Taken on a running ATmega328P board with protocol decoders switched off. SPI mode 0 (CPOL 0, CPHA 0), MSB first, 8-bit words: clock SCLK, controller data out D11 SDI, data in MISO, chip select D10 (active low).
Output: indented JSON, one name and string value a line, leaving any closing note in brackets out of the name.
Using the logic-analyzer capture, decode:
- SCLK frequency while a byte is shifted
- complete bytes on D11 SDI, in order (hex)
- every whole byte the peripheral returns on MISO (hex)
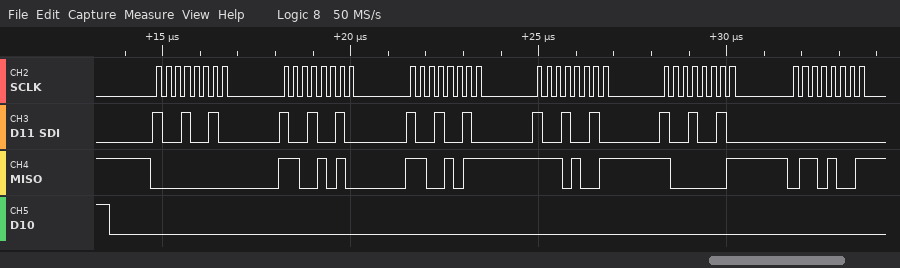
{
  "SCLK frequency while a byte is shifted": "4 MHz",
  "complete bytes on D11 SDI, in order": "92 92 92 92 92 00",
  "every whole byte the peripheral returns on MISO": "00 CA CB E9 81 69"
}
